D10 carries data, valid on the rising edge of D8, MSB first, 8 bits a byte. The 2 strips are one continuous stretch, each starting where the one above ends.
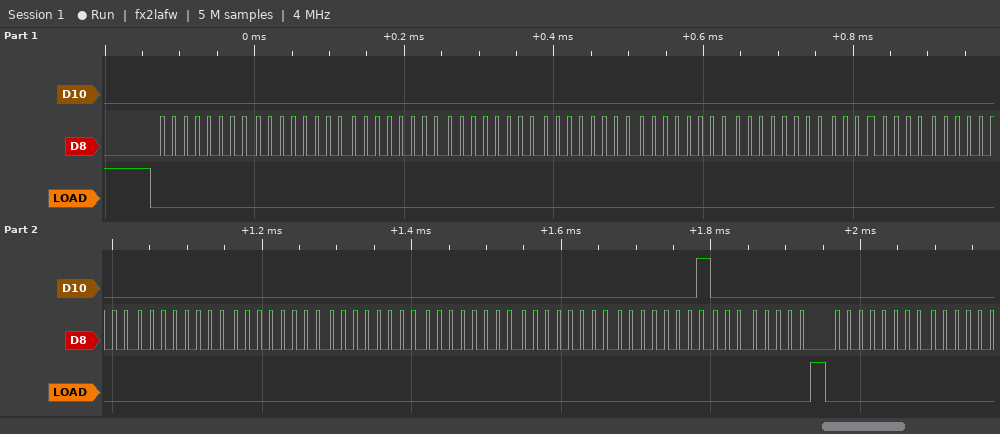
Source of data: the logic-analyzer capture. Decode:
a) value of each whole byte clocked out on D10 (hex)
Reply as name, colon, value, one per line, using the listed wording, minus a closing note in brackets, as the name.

value of each whole byte clocked out on D10: 00 00 00 00 00 00 00 00 00 00 00 00 00 00 01 00 00
